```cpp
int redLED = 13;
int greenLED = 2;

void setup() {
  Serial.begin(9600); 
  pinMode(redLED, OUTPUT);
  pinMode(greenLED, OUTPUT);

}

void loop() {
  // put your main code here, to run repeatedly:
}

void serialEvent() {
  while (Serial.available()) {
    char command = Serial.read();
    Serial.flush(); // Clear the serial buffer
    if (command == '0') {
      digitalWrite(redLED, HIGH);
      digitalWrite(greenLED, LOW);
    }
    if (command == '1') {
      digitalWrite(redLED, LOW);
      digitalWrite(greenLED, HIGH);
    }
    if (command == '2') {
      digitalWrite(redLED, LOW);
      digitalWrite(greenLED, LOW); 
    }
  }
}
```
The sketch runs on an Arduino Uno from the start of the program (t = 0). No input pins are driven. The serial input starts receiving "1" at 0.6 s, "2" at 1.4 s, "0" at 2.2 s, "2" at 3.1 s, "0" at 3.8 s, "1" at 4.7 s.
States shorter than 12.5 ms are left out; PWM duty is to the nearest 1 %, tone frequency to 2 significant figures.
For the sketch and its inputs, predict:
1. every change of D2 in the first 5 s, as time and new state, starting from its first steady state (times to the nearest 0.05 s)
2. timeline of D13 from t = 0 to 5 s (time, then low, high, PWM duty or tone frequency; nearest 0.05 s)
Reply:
0 s low; 0.6 s high; 1.4 s low; 4.7 s high
0 s low; 2.2 s high; 3.1 s low; 3.8 s high; 4.7 s low
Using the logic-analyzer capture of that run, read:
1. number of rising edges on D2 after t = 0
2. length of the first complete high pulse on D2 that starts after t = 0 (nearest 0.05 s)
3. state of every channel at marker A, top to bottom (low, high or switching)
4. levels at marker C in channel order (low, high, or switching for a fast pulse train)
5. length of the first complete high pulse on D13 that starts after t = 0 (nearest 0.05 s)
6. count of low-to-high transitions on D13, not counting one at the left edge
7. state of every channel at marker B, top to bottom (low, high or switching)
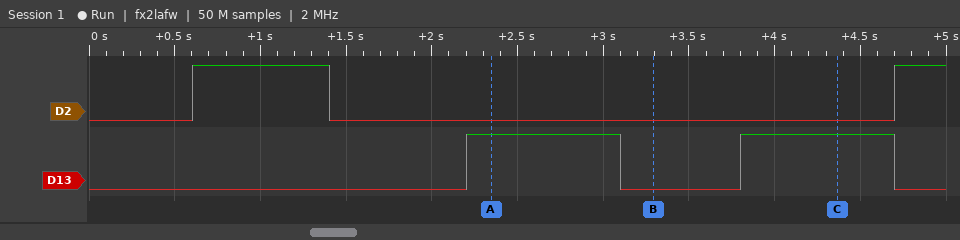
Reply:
2
0.80 s
D2 low, D13 high
D2 low, D13 high
0.90 s
2
D2 low, D13 low
